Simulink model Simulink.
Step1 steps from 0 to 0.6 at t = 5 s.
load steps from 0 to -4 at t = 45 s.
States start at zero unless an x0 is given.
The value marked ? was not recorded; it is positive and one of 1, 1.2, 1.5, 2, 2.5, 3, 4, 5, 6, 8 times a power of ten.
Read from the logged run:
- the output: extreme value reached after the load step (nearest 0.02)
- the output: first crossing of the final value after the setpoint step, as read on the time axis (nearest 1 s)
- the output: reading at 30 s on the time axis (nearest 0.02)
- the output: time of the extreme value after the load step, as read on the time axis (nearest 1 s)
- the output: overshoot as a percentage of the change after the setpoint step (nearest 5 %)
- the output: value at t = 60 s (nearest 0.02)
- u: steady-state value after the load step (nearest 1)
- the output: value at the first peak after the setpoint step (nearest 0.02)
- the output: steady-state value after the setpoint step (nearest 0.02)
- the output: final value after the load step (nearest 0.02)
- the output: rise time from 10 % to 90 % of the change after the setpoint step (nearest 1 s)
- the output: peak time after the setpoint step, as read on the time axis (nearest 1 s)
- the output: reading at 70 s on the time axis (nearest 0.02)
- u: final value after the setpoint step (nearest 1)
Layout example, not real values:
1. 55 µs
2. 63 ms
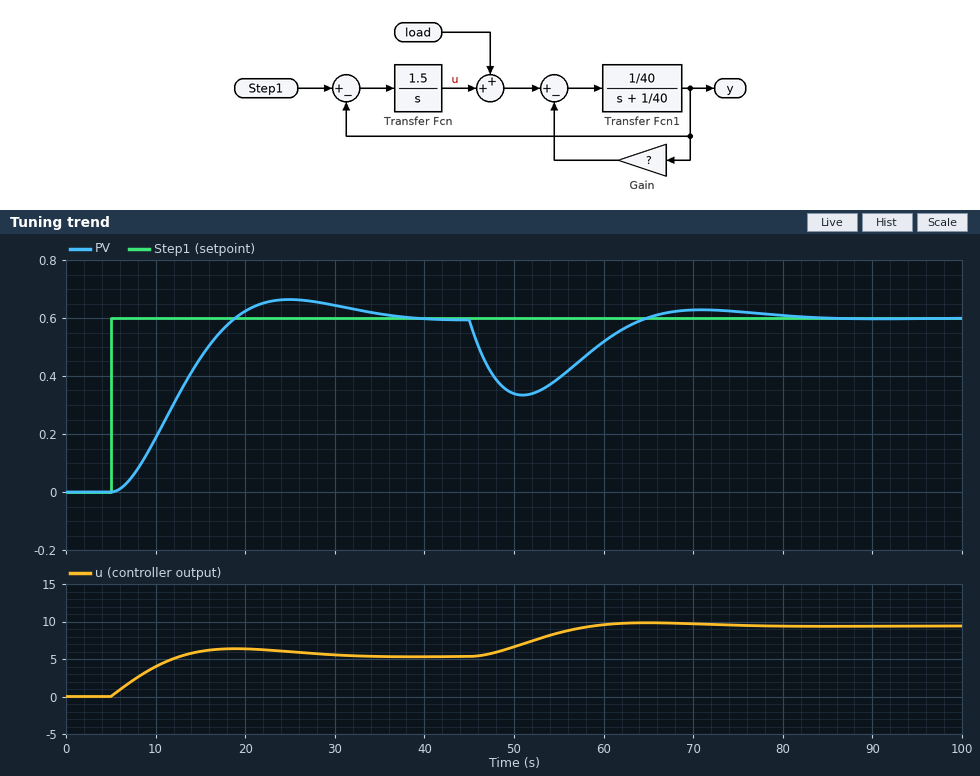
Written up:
1. 0.34
2. 19 s
3. 0.64
4. 51 s
5. 10 %
6. 0.52
7. 9
8. 0.66
9. 0.60
10. 0.60
11. 9 s
12. 25 s
13. 0.62
14. 5
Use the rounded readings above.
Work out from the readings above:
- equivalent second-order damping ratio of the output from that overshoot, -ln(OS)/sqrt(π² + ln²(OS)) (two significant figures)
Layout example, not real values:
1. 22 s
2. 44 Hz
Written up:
1. 0.59
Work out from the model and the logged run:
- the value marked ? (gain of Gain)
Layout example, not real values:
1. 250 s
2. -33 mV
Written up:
1. 8
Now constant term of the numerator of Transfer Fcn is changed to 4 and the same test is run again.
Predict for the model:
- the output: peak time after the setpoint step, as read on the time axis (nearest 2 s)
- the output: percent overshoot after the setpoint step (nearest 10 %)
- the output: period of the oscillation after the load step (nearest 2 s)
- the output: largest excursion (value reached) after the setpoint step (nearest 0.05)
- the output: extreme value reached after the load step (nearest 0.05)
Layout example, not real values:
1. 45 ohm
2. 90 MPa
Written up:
1. 16 s
2. 30 %
3. 22 s
4. 0.80
5. 0.40
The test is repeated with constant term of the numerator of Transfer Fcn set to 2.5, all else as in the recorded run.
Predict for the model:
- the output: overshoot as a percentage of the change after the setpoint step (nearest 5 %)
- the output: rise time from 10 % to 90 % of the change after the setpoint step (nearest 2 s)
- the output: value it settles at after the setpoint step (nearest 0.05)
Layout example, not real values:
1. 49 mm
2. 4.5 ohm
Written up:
1. 20 %
2. 6 s
3. 0.60
